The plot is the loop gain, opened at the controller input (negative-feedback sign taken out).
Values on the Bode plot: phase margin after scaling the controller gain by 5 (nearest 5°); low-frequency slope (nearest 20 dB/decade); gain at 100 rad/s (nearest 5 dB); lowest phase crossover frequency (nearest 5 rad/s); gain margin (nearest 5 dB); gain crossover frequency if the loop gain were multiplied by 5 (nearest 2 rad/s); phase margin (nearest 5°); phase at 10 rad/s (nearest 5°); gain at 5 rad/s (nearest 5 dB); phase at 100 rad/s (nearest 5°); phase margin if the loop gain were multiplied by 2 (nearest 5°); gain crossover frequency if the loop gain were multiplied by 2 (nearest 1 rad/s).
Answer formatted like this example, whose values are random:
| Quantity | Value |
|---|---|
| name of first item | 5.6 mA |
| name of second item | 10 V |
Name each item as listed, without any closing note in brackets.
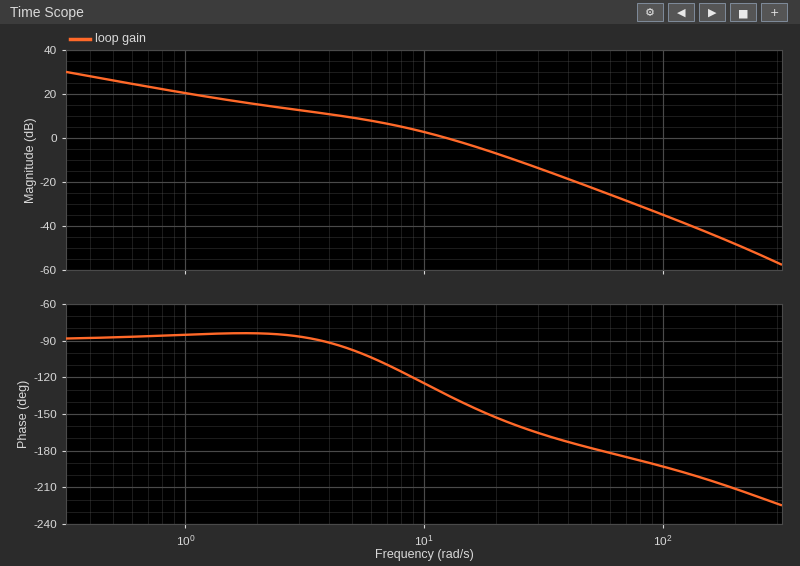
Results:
| Quantity | Value |
|---|---|
| phase margin after scaling the controller gain by 5 | 15° |
| low-frequency slope | -20 dB/decade |
| gain at 100 rad/s | -35 dB |
| lowest phase crossover frequency | 55 rad/s |
| gain margin | 25 dB |
| gain crossover frequency if the loop gain were multiplied by 5 | 30 rad/s |
| phase margin | 45° |
| phase at 10 rad/s | -125° |
| gain at 5 rad/s | 10 dB |
| phase at 100 rad/s | -195° |
| phase margin if the loop gain were multiplied by 2 | 30° |
| gain crossover frequency if the loop gain were multiplied by 2 | 19 rad/s |
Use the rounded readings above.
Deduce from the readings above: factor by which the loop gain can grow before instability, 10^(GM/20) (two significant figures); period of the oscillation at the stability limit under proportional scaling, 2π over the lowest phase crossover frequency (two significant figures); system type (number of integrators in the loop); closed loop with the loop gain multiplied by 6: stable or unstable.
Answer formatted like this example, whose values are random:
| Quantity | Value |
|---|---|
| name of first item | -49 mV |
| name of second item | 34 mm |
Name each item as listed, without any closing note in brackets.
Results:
| Quantity | Value |
|---|---|
| factor by which the loop gain can grow before instability, 10^(GM/20) | 18 |
| period of the oscillation at the stability limit under proportional scaling, 2π over the lowest phase crossover frequency | 0.11 s |
| system type | 1 |
| closed loop with the loop gain multiplied by 6: stable or unstable | stable |
